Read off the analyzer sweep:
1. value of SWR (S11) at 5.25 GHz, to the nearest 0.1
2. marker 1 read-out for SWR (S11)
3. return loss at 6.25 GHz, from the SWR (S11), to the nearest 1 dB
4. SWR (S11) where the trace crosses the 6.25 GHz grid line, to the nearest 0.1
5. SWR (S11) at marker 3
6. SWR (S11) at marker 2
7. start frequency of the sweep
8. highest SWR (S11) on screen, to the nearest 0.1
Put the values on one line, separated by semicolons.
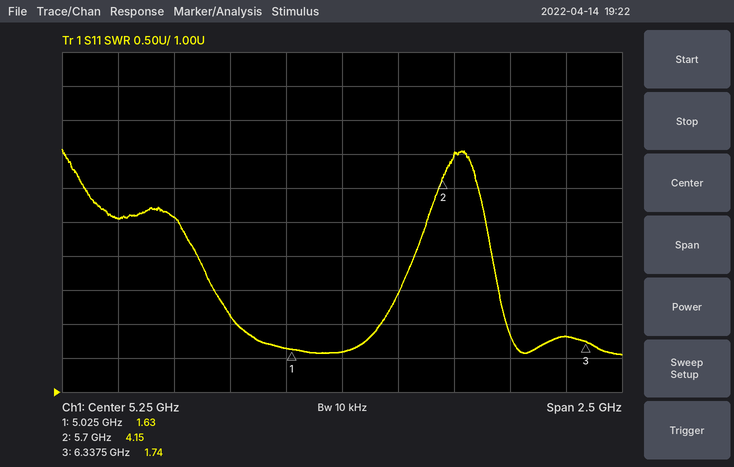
1.6; 1.63; 11 dB; 1.8; 1.74; 4.15; 4 GHz; 4.6
